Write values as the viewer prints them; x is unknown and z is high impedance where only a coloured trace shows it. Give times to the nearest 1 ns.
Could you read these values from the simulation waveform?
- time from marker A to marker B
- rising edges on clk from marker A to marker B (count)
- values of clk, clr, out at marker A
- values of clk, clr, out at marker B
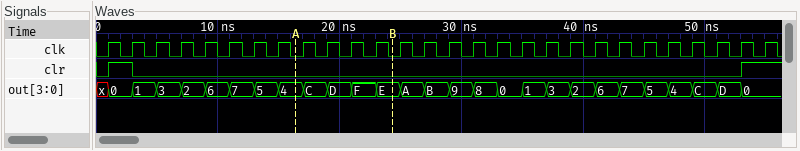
8 ns
4
clk=0, clr=0, out=4
clk=0, clr=0, out=E
